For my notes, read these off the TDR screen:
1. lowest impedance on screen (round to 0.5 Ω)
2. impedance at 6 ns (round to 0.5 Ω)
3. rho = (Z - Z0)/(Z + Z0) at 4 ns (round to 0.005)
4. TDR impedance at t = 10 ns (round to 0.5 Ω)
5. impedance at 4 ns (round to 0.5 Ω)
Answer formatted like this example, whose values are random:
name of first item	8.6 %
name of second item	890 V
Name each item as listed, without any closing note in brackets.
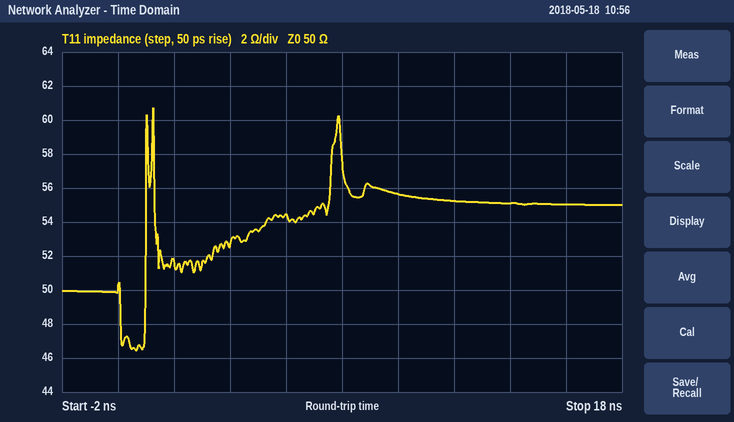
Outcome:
lowest impedance on screen	46.5 Ω
impedance at 6 ns	54.5 Ω
rho = (Z - Z0)/(Z + Z0) at 4 ns	+0.025
TDR impedance at t = 10 ns	55.5 Ω
impedance at 4 ns	52.5 Ω
